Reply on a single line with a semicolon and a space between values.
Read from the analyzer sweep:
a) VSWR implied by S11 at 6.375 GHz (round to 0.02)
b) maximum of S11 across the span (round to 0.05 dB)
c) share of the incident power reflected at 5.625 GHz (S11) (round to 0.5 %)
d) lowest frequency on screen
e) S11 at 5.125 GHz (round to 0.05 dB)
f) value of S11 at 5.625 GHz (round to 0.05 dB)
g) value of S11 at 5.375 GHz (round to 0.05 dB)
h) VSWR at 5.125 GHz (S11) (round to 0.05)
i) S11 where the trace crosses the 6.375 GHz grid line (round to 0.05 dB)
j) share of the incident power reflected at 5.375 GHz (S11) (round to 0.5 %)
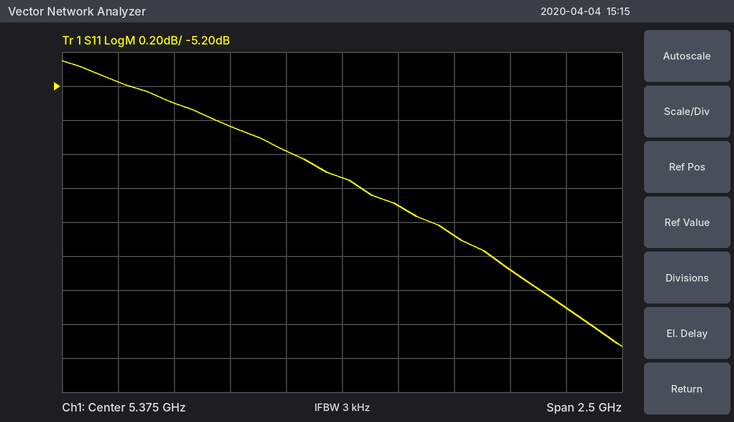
2.80; -5.05 dB; 25.5 %; 4.125 GHz; -5.60 dB; -5.90 dB; -5.75 dB; 3.20; -6.50 dB; 26.5 %
